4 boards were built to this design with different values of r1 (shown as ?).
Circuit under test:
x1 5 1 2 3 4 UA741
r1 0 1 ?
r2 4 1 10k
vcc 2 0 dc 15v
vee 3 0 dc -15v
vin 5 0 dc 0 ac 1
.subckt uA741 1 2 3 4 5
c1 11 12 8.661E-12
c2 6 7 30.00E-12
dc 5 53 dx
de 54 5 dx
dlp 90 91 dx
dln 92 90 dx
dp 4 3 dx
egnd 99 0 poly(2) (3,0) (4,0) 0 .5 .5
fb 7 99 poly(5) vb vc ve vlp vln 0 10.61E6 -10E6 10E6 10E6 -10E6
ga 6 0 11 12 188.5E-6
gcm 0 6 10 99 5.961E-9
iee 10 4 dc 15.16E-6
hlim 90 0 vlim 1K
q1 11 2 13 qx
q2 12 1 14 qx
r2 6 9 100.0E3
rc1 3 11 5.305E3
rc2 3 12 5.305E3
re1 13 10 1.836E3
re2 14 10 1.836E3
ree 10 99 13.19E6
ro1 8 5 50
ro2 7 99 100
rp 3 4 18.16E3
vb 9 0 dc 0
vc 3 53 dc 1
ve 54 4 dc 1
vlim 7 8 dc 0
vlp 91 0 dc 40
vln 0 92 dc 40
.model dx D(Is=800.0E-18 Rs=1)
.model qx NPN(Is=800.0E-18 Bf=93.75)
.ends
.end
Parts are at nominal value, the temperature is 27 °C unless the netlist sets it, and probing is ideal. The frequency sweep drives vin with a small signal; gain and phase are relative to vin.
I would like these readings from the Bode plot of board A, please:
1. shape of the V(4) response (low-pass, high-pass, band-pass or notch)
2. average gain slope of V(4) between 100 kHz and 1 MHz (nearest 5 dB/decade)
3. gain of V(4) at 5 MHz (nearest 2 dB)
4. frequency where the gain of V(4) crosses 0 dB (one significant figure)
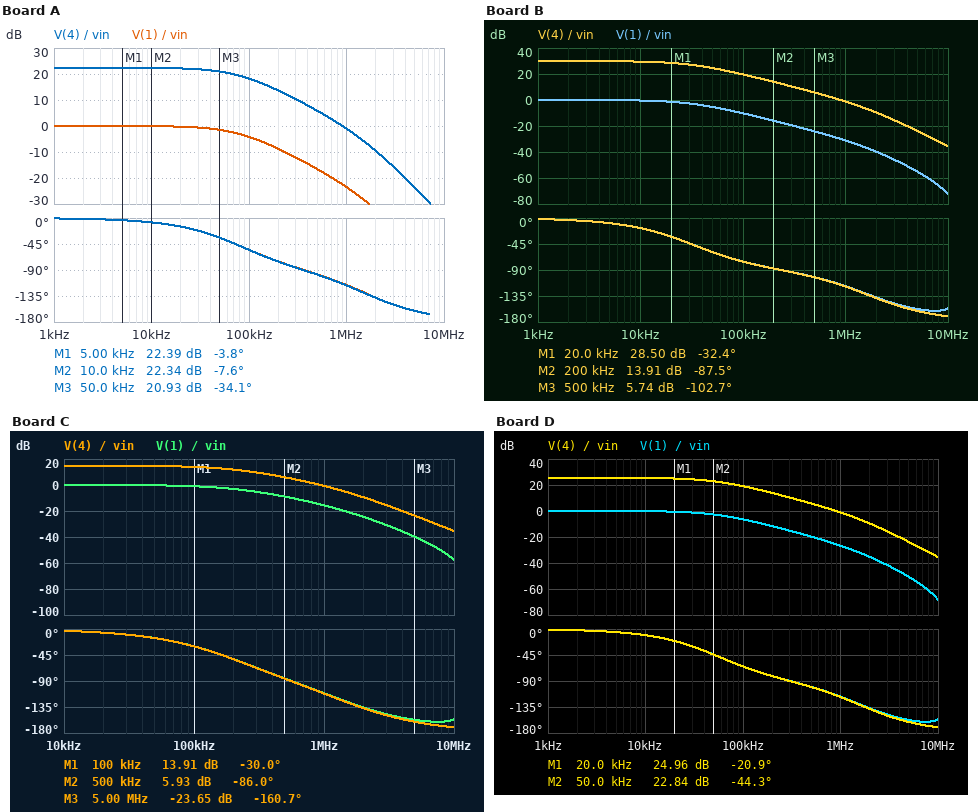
low-pass
-20 dB/decade
-24 dB
900 kHz
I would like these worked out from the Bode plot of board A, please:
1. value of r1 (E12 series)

820 Ω
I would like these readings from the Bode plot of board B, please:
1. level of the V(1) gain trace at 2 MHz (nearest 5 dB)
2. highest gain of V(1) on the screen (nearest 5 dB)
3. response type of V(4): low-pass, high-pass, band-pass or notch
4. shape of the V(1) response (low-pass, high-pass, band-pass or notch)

-40 dB
0 dB
low-pass
low-pass
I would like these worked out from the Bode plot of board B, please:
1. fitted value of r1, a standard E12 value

330 Ω
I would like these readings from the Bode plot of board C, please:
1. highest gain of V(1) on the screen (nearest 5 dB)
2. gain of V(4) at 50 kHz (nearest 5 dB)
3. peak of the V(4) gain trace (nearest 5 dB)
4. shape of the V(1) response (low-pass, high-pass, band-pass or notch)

0 dB
15 dB
15 dB
low-pass
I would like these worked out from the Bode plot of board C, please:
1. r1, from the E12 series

2.2 kΩ
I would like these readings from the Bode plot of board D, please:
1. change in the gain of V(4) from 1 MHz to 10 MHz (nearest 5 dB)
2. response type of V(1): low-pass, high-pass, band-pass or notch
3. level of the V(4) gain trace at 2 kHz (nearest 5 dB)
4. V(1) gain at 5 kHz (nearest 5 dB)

-35 dB
low-pass
25 dB
0 dB
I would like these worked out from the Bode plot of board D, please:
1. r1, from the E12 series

560 Ω
